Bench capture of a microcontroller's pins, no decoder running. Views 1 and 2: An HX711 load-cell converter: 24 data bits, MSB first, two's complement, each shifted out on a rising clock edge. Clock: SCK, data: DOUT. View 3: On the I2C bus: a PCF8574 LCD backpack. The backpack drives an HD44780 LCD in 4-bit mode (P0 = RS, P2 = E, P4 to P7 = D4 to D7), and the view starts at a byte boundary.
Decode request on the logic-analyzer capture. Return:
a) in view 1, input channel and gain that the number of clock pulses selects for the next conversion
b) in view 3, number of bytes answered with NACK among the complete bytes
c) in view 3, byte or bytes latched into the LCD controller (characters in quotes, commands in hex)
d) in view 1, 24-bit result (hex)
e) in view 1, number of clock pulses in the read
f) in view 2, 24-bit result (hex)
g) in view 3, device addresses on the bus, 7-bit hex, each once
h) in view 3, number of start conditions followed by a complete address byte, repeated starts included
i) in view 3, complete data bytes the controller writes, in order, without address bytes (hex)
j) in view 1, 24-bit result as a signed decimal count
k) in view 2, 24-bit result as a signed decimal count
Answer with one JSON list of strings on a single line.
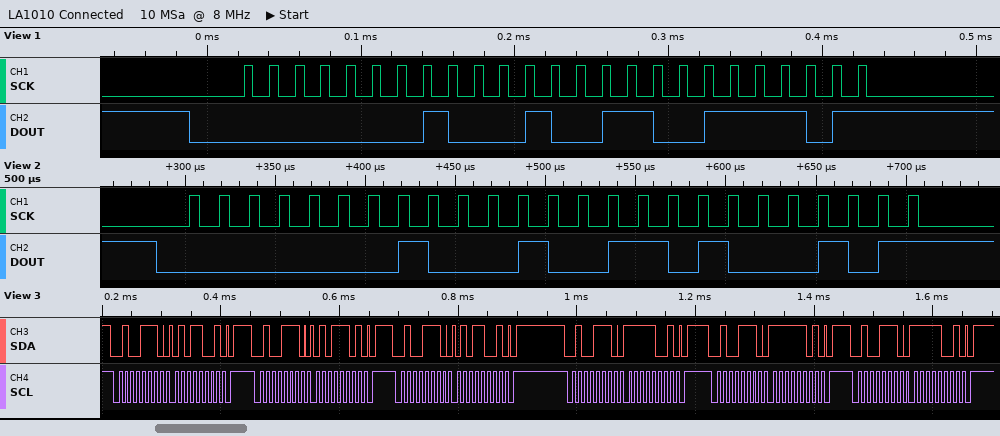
["channel A, gain 128", "0", "'_'", "0x01133D", "25", "0x011345", "0x27", "6", "59 5D 59 F9 FD F9", "70461", "70469"]
